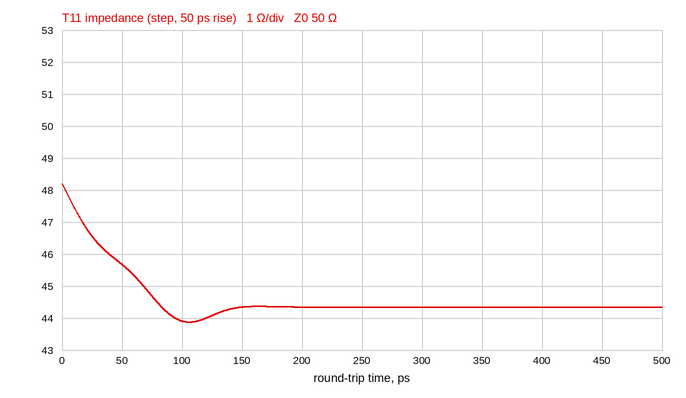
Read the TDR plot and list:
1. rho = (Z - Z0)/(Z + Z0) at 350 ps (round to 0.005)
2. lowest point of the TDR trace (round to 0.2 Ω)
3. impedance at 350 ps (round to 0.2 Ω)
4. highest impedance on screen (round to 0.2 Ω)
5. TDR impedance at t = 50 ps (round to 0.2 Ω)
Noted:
-0.060
43.8 Ω
44.4 Ω
48.2 Ω
45.6 Ω
